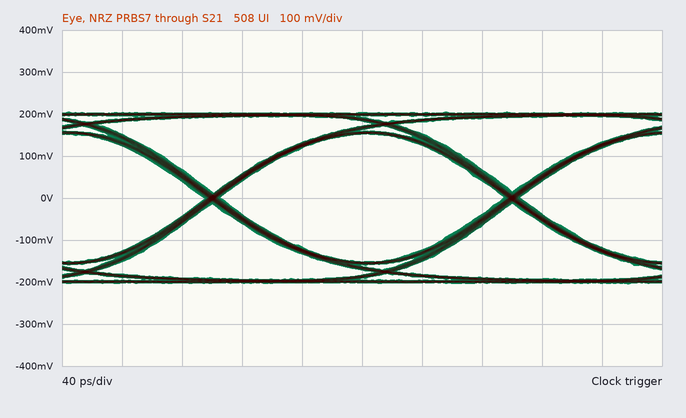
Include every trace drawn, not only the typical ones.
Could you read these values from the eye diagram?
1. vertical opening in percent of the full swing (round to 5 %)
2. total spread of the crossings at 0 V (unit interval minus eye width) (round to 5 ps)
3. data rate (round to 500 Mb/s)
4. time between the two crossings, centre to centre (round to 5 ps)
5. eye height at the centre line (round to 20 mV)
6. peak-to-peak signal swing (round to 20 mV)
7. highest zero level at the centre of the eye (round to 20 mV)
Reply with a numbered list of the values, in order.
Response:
1. 75 %
2. 10 ps
3. 5.0 Gb/s
4. 200 ps
5. 300 mV
6. 400 mV
7. -160 mV
